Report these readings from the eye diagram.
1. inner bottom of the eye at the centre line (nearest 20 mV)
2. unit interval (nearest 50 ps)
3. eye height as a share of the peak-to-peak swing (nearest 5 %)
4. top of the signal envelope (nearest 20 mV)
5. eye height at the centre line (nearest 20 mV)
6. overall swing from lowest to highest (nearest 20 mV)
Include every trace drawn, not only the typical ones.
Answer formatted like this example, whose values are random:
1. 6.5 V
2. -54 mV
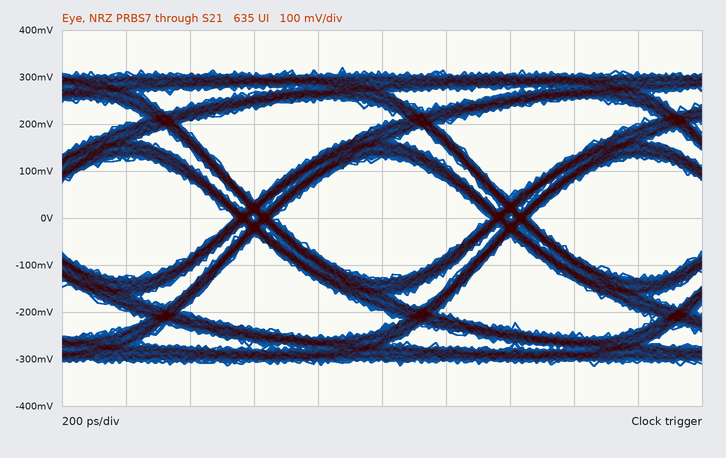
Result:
1. -120 mV
2. 800 ps
3. 40 %
4. 320 mV
5. 260 mV
6. 640 mV
